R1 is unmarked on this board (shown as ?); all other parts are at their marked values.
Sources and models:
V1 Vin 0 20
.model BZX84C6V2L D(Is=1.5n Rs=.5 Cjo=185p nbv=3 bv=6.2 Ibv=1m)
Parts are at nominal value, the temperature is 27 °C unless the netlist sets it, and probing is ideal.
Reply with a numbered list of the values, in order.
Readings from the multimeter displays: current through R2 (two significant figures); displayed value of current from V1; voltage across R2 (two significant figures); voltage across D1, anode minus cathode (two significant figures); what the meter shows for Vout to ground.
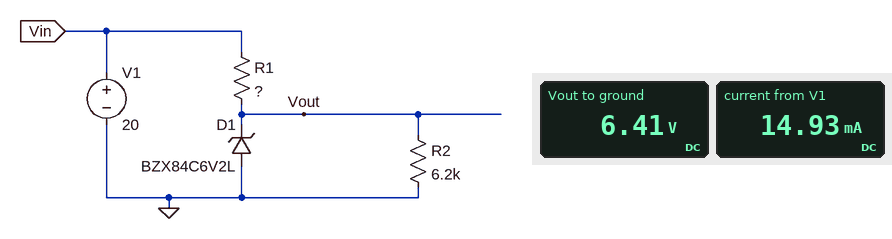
1. 1.0 mA
2. 14.93 mA
3. 6.4 V
4. -6.4 V
5. 6.41 V
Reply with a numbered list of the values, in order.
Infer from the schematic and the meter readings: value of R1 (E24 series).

1. 910 Ω
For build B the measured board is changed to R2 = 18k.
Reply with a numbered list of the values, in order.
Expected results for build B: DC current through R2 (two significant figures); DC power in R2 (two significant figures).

1. 360 µA
2. 2.3 mW
